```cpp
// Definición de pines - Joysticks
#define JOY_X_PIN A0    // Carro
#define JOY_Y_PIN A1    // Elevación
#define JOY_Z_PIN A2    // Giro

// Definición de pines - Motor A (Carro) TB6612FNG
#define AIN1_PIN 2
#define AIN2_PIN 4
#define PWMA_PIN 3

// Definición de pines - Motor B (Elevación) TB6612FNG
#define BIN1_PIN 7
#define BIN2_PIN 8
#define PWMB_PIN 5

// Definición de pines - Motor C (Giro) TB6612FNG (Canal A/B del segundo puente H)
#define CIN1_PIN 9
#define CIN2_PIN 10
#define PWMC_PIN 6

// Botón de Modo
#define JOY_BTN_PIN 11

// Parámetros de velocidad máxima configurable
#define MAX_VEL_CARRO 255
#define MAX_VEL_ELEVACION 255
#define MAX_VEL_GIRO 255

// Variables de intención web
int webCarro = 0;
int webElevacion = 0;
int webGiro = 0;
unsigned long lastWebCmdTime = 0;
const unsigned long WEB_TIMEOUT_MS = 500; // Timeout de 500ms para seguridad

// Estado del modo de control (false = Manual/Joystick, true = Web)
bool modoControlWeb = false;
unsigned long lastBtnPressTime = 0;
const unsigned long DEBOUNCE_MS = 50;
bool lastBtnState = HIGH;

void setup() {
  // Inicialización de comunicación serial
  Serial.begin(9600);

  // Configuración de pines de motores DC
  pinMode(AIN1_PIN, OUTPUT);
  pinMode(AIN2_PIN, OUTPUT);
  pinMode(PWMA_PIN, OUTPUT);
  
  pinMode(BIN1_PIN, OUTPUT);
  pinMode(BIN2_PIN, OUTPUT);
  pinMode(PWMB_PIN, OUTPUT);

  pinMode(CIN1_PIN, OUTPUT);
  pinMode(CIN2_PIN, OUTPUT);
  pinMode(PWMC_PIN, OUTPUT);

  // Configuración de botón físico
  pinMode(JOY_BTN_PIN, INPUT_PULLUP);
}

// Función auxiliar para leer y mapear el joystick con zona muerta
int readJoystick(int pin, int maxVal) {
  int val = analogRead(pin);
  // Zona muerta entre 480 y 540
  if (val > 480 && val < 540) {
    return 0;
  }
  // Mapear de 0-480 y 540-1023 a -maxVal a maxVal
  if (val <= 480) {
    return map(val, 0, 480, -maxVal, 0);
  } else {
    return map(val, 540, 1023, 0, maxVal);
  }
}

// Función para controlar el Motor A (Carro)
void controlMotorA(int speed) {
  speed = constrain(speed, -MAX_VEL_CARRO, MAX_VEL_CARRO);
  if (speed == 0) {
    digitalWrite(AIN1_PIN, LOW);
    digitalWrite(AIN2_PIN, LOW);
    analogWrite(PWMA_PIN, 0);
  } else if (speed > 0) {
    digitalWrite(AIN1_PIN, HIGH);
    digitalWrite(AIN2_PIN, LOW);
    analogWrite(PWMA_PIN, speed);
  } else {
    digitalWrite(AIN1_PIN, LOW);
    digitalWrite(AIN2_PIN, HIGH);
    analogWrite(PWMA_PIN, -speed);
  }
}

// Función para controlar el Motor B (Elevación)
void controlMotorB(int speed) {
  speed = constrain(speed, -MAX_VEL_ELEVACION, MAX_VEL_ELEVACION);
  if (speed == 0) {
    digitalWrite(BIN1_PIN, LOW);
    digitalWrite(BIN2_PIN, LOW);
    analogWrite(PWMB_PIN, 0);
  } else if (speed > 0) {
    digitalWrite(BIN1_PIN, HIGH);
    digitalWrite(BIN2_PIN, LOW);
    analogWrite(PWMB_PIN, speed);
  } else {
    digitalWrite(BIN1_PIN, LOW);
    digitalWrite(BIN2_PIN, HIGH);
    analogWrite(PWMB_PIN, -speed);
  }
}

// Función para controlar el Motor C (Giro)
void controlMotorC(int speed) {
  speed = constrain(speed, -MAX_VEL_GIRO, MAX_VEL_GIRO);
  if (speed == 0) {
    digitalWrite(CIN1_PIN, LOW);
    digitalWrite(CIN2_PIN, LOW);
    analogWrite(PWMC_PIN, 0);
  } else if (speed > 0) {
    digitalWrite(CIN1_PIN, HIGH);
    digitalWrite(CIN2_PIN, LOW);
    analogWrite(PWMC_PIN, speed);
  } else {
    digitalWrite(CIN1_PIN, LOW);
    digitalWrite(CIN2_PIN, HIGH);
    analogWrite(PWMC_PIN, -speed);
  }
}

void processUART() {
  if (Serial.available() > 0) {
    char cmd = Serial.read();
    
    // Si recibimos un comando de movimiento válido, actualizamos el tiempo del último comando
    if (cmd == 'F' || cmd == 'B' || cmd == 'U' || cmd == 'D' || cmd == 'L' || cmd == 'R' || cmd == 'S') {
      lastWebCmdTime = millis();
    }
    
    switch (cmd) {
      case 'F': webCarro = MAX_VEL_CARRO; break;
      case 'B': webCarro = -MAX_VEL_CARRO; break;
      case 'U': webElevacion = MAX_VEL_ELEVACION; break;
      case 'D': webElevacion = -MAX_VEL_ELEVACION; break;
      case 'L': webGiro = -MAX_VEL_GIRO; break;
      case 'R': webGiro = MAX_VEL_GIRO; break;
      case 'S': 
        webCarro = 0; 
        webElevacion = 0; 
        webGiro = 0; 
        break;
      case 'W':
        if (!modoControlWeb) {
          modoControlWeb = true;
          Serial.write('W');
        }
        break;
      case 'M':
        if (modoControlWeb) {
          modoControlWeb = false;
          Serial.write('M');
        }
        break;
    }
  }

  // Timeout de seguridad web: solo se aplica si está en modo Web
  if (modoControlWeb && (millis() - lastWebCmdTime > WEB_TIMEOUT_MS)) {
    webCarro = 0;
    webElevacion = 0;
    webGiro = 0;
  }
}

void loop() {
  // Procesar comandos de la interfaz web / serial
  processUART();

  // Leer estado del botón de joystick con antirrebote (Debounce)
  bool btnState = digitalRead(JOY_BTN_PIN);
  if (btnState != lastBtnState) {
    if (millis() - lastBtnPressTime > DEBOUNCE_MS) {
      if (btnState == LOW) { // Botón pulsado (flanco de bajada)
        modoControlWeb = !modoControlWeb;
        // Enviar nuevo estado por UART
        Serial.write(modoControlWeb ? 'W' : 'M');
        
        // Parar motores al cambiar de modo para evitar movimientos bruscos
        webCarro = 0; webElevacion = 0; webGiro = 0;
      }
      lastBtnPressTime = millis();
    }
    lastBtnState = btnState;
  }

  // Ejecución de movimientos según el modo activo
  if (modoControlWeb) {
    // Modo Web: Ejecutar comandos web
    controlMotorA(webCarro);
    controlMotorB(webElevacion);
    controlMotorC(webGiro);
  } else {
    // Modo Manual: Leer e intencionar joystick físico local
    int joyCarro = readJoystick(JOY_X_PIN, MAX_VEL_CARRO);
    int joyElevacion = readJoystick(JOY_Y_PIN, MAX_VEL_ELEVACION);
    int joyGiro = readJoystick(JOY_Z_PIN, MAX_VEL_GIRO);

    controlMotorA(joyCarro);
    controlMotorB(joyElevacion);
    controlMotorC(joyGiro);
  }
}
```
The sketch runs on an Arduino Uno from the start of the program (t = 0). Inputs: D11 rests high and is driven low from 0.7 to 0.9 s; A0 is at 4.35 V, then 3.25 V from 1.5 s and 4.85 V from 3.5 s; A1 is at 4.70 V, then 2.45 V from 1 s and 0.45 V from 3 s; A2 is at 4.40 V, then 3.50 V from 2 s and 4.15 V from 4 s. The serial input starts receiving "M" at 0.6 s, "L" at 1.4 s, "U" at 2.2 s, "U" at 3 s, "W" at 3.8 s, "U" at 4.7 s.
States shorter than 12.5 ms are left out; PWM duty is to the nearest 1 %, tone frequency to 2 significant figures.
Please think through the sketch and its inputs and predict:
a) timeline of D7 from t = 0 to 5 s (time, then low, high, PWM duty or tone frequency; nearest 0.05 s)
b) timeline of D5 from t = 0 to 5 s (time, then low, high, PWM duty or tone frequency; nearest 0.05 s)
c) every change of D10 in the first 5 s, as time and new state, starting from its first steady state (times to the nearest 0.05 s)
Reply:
0 s high; 0.7 s low; 2.2 s high; 2.7 s low; 3 s high; 3.5 s low; 4.7 s high
0 s PWM 87 %; 0.7 s low; 2.2 s high; 2.7 s low; 3 s high; 3.5 s low; 4.7 s high
0 s low; 1.4 s high; 1.9 s low
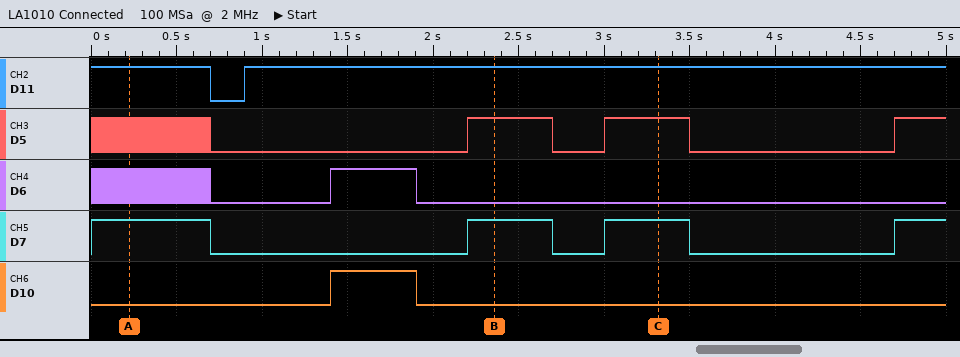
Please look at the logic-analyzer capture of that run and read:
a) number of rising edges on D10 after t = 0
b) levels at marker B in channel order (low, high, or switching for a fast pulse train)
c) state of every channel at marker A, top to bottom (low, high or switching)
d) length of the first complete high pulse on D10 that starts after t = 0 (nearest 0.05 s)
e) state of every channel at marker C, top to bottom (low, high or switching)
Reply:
1
D11 high, D5 high, D6 low, D7 high, D10 low
D11 high, D5 switching, D6 switching, D7 high, D10 low
0.50 s
D11 high, D5 high, D6 low, D7 high, D10 low
